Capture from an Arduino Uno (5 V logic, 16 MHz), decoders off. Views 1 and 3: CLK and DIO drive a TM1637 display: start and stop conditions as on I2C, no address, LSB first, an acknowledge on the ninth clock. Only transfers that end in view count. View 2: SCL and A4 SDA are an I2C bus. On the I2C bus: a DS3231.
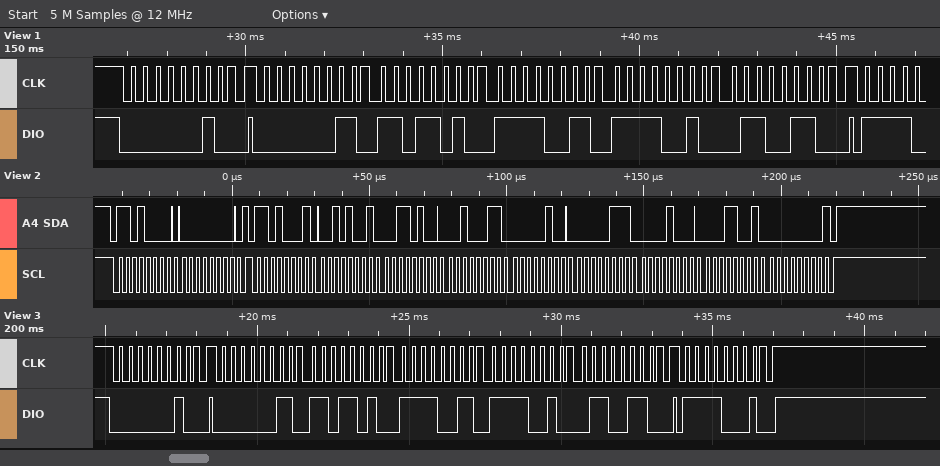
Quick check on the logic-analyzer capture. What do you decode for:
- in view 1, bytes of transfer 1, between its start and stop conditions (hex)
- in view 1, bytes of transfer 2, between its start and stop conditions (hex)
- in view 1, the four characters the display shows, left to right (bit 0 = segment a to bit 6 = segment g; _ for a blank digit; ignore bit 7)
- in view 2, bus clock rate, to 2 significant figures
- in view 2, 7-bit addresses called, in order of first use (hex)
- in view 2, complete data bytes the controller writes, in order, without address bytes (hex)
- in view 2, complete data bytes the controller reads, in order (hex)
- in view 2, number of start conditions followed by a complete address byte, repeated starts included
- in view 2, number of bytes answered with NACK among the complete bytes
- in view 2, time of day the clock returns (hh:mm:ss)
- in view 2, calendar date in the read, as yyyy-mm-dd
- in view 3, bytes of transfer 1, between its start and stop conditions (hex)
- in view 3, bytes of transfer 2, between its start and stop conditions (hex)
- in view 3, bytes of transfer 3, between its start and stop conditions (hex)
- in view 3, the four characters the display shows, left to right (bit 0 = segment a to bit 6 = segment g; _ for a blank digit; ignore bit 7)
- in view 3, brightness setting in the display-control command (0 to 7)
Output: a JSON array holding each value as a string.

["40", "C0 5B CF 4F 66", "2334", "400 kHz", "0x68", "00", "29 34 23 04 07 08 19 00", "2", "1", "23:34:29", "2019-08-07", "40", "C0 5B CF 4F 66", "8F", "2334", "7"]
